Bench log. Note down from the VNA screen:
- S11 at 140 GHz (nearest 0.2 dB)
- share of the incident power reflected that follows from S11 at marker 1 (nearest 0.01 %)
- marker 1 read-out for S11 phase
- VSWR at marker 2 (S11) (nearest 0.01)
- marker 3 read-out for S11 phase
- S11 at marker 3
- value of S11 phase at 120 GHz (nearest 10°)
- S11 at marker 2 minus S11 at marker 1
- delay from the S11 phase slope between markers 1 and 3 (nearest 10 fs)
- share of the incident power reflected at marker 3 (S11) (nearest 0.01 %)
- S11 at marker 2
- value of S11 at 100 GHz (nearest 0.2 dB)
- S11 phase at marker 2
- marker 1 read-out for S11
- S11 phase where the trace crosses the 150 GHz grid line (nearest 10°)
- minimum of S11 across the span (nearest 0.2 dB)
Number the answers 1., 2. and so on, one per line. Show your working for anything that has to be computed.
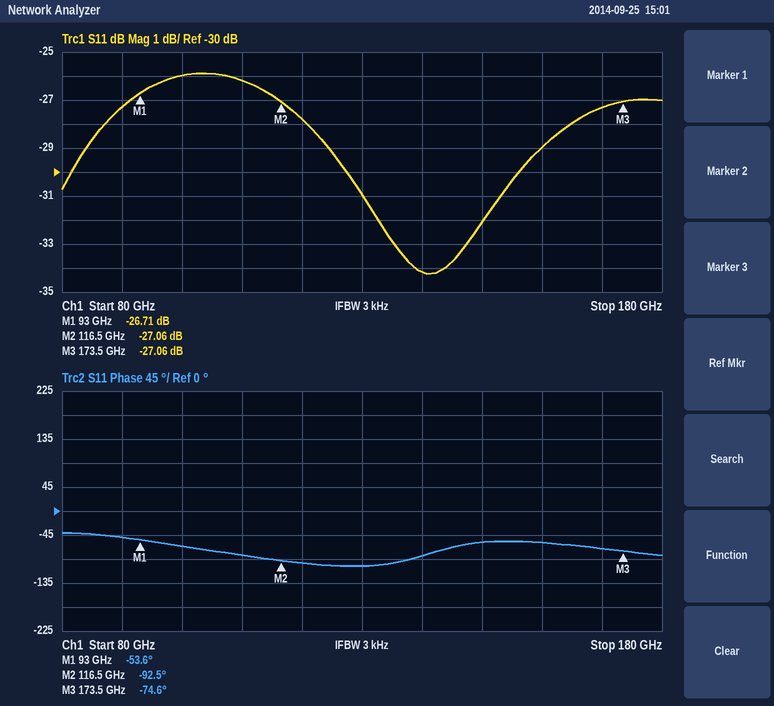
1. -34.2 dB
2. 10^(-26.71/10) ≈ 0.21 %
3. -53.6°
4. (1 + 0.0444)/(1 − 0.0444) ≈ 1.09
5. -74.6°
6. -27.06 dB
7. -100°
8. -27.06 − (-26.71) = -0.35 dB
9. −(-74.6° − (-53.6°))/(360° × 80.5 GHz) ≈ 725 fs, so 720 fs to the nearest 10 fs
10. 10^(-27.06/10) ≈ 0.20 %
11. -27.06 dB
12. -26.0 dB
13. -92.5°
14. -26.71 dB
15. -60°
16. -34.2 dB
